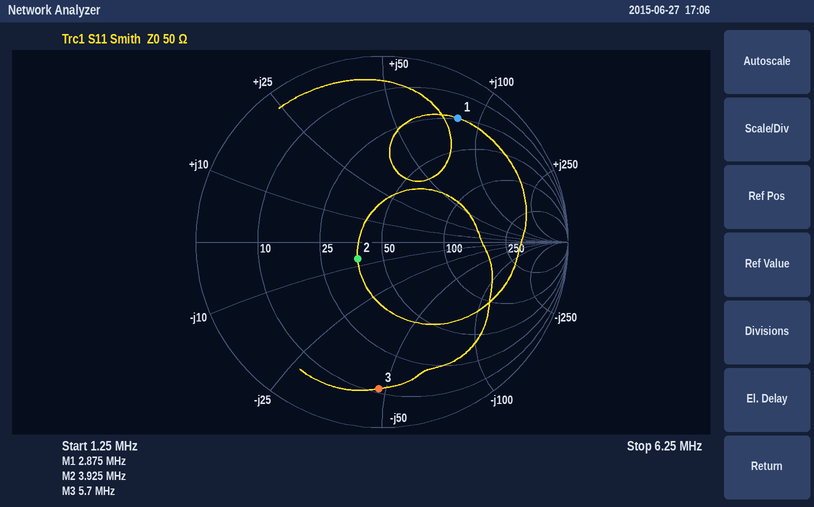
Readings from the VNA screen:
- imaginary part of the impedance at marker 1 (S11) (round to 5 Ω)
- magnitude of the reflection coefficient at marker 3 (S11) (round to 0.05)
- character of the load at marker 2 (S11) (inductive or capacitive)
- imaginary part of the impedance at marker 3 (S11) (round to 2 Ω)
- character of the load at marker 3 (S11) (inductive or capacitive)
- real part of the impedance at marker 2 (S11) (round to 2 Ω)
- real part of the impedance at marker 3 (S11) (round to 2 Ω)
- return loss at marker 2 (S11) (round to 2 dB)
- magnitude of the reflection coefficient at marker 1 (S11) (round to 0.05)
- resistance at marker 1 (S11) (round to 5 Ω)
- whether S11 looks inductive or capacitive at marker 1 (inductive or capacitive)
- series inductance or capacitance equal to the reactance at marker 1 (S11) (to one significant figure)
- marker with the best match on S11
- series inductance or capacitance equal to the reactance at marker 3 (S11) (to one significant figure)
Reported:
+85 Ω
0.80
capacitive
-48 Ω
capacitive
38 Ω
12 Ω
16 dB
0.80
25 Ω
inductive
5 µH
marker 2
600 pF
